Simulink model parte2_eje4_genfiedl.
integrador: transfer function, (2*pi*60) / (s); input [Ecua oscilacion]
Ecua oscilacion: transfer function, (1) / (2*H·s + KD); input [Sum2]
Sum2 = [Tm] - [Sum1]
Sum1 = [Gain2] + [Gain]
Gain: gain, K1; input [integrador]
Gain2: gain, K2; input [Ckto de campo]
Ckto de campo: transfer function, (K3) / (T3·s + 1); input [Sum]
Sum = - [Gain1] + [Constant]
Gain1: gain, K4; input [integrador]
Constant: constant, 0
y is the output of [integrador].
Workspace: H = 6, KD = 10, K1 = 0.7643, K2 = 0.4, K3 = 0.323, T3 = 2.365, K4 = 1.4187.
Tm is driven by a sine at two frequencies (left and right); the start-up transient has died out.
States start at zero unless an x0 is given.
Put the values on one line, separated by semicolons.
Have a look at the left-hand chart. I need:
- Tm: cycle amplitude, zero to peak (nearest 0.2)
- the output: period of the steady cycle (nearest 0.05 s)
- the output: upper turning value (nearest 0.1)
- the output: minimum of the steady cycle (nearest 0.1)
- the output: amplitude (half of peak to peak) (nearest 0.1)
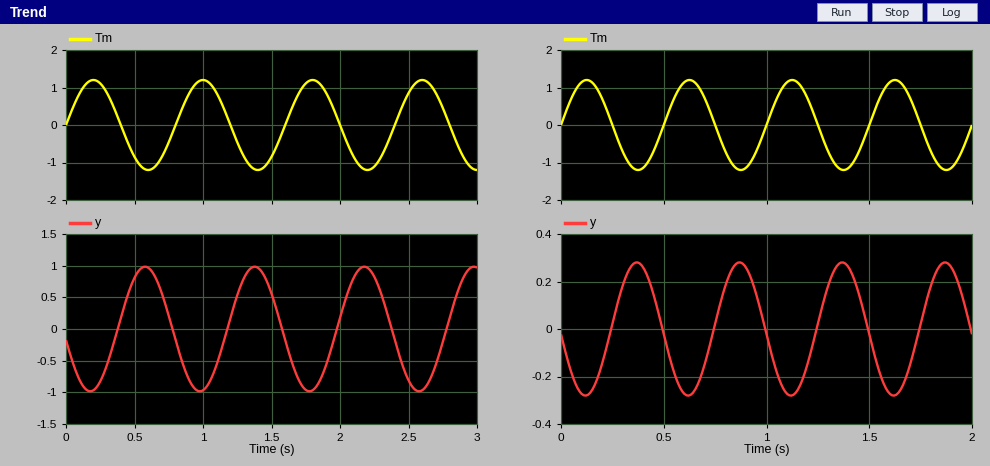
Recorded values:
1.2; 0.80 s; 1.0; -1.0; 1.0
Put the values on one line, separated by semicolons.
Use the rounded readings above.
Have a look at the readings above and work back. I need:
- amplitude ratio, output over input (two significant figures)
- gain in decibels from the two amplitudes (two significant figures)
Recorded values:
0.83; -1.6 dB
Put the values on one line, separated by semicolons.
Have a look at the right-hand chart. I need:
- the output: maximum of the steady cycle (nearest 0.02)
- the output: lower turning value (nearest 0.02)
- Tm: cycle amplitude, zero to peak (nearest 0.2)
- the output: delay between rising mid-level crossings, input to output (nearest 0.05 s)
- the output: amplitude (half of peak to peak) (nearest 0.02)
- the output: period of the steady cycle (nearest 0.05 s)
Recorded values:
0.28; -0.28; 1.2; 0.25 s; 0.28; 0.50 s
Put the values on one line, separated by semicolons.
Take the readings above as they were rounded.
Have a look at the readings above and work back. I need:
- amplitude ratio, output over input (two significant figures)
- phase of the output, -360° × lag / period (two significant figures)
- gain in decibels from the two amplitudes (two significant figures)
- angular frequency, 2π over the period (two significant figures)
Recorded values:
0.23; -180°; -13 dB; 13 rad/s
